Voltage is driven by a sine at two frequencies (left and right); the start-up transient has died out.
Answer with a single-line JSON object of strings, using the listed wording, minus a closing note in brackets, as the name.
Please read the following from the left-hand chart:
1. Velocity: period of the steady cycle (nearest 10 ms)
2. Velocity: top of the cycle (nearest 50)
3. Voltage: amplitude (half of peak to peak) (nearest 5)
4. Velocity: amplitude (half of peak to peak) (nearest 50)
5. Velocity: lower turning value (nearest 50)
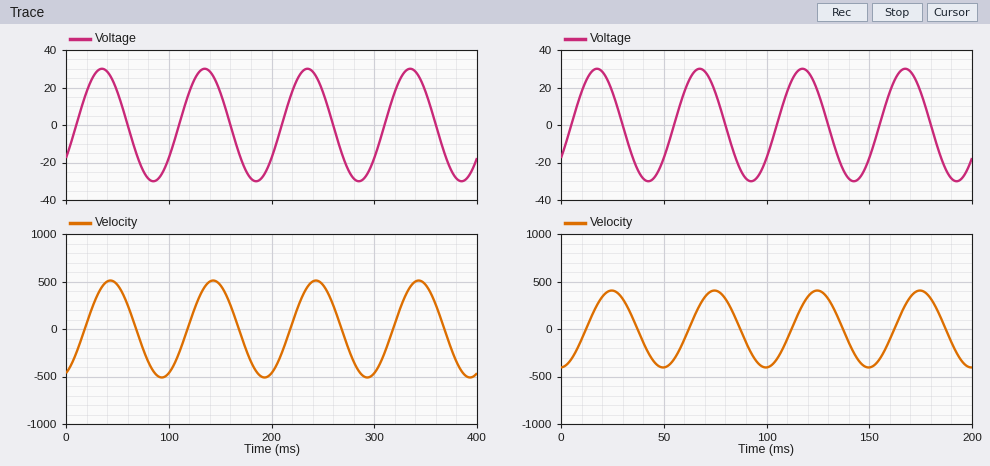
{"Velocity: period of the steady cycle": "100 ms", "Velocity: top of the cycle": "500", "Voltage: amplitude (half of peak to peak)": "30", "Velocity: amplitude (half of peak to peak)": "500", "Velocity: lower turning value": "-500"}
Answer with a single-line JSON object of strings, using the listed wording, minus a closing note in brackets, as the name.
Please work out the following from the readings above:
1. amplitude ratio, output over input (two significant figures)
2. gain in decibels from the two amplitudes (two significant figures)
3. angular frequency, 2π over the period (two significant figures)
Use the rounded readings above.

{"amplitude ratio, output over input": "17", "gain in decibels from the two amplitudes": "24 dB", "angular frequency, 2π over the period": "0.063 rad/ms"}
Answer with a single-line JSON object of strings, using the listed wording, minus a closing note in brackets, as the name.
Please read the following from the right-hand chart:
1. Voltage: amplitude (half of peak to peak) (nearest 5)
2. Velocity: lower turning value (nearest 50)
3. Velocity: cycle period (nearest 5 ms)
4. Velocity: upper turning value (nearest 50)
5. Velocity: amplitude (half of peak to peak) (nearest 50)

{"Voltage: amplitude (half of peak to peak)": "30", "Velocity: lower turning value": "-400", "Velocity: cycle period": "50 ms", "Velocity: upper turning value": "400", "Velocity: amplitude (half of peak to peak)": "400"}
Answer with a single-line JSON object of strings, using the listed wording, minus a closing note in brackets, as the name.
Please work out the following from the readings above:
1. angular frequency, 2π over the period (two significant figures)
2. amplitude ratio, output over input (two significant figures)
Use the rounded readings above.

{"angular frequency, 2π over the period": "0.13 rad/ms", "amplitude ratio, output over input": "13"}
